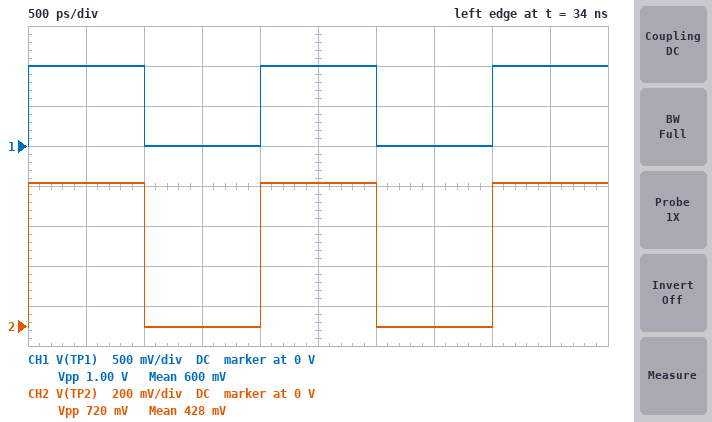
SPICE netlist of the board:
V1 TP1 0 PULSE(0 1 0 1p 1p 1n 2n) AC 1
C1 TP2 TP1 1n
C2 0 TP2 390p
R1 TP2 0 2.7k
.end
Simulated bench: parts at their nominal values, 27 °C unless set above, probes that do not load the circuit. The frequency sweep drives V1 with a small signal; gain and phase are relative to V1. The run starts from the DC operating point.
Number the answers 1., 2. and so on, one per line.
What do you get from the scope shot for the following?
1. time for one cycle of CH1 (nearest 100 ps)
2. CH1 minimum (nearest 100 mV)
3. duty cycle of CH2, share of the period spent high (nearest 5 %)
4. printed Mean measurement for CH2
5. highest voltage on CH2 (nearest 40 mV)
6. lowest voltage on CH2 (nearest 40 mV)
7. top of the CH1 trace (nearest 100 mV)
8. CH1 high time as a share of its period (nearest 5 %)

1. 2.0 ns
2. 0 V
3. 50 %
4. 428 mV
5. 720 mV
6. 0 V
7. 1.0 V
8. 50 %
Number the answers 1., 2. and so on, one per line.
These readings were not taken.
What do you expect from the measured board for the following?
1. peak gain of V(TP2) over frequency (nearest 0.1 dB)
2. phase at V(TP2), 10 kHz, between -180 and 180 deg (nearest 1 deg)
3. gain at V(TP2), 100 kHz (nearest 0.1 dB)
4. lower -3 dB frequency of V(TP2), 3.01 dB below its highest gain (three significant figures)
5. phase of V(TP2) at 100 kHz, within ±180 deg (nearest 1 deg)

1. -2.9 dB
2. 77 deg
3. -3.6 dB
4. 42.4 kHz
5. 23 deg
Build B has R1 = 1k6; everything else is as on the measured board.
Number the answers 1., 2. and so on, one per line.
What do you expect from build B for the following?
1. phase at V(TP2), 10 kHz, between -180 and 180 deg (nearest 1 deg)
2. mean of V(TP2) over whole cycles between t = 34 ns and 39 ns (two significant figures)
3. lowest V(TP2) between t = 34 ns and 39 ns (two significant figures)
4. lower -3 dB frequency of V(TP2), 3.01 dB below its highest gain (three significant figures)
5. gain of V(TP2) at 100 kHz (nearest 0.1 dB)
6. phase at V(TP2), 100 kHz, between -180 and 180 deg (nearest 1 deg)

1. 82 deg
2. 350 mV
3. -6.1 mV
4. 71.6 kHz
5. -4.7 dB
6. 36 deg
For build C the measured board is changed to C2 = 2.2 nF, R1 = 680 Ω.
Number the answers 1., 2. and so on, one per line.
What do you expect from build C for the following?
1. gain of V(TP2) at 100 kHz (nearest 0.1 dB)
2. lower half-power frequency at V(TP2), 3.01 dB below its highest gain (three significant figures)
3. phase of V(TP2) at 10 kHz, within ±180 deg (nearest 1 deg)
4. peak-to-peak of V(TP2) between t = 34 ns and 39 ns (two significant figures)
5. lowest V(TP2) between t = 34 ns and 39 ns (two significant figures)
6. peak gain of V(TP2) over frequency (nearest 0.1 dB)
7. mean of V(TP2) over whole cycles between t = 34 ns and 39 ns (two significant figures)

1. -12.0 dB
2. 73.1 kHz
3. 82 deg
4. 310 mV
5. -2.7 mV
6. -10.1 dB
7. 150 mV
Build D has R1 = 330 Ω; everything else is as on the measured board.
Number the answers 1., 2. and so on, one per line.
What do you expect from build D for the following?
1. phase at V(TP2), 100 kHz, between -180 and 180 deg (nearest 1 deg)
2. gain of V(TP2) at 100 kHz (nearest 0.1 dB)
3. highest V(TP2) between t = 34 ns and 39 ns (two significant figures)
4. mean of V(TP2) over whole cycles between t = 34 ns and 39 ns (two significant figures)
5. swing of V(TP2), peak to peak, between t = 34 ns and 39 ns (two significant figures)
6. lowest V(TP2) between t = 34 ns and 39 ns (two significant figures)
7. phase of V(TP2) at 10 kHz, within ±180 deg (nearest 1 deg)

1. 74 deg
2. -14.0 dB
3. 690 mV
4. 330 mV
5. 720 mV
6. -29 mV
7. 88 deg
